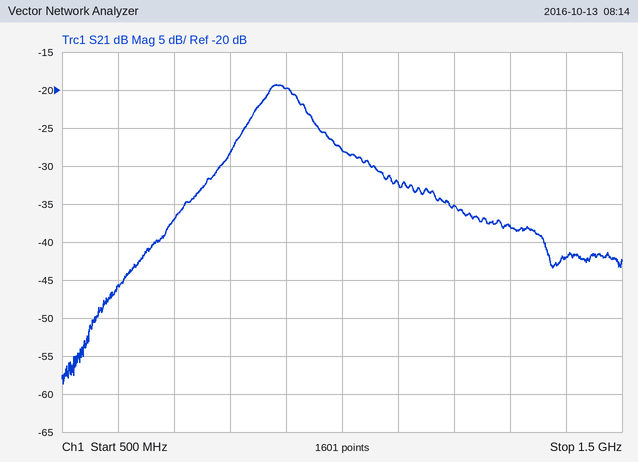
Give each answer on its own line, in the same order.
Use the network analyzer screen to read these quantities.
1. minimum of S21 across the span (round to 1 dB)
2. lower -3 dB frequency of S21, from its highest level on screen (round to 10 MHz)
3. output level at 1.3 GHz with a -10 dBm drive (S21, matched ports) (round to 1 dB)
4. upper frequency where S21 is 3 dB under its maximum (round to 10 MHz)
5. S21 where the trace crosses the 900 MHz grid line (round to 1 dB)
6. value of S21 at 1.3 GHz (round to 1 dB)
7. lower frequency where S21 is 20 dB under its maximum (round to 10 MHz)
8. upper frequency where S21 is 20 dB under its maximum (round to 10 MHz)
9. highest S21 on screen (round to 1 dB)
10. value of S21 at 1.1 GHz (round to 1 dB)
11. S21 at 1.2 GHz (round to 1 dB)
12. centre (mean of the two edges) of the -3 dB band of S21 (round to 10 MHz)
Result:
-59 dB
850 MHz
-48 dBm
930 MHz
-20 dB
-38 dB
680 MHz
1.36 GHz
-19 dB
-32 dB
-35 dB
890 MHz
